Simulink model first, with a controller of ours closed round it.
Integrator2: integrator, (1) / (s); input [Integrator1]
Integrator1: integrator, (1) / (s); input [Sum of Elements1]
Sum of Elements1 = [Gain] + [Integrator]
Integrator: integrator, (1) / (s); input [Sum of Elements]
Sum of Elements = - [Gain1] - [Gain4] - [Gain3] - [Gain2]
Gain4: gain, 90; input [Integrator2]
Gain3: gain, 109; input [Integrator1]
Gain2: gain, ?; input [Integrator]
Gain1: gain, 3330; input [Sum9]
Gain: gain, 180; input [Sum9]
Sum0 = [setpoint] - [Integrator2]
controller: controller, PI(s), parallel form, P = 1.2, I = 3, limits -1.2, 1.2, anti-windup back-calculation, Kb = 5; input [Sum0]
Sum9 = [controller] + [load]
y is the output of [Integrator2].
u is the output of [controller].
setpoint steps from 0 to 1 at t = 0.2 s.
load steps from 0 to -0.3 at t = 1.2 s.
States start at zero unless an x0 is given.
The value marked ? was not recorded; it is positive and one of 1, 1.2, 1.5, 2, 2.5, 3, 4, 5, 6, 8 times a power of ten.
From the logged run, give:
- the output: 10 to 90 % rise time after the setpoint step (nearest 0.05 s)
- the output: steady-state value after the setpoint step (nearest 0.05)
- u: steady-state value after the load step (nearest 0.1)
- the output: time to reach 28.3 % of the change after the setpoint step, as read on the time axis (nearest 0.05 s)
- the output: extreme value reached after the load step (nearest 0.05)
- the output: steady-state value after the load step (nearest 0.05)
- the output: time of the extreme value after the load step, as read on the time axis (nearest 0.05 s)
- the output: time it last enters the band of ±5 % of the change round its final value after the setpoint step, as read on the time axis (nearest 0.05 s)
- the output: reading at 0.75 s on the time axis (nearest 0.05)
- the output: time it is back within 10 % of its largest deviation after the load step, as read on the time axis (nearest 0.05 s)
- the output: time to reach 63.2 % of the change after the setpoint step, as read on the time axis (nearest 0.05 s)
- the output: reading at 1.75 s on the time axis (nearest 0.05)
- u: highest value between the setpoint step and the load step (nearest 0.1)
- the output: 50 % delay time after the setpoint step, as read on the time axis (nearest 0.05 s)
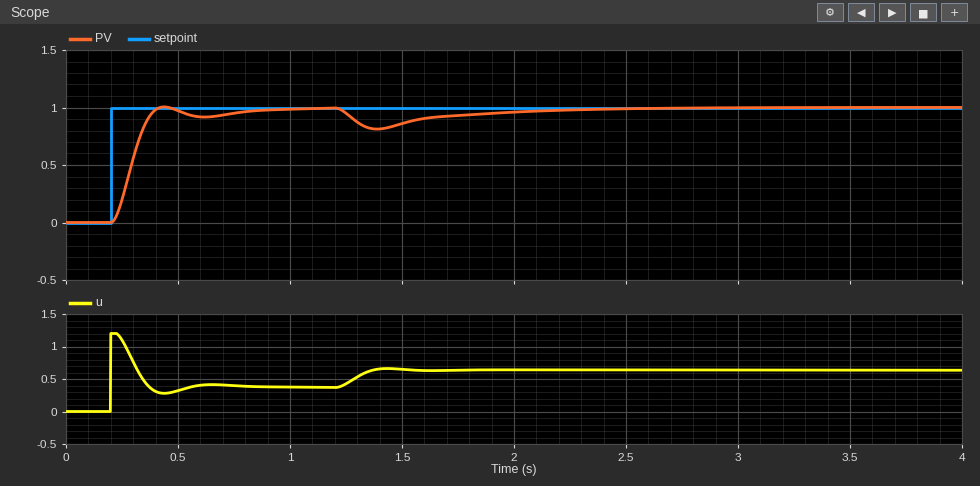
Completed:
0.15 s
1.00
0.6
0.25 s
0.80
1.00
1.40 s
0.75 s
0.95
2.30 s
0.30 s
0.95
1.2
0.30 s
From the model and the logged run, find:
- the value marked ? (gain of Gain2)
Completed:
20
